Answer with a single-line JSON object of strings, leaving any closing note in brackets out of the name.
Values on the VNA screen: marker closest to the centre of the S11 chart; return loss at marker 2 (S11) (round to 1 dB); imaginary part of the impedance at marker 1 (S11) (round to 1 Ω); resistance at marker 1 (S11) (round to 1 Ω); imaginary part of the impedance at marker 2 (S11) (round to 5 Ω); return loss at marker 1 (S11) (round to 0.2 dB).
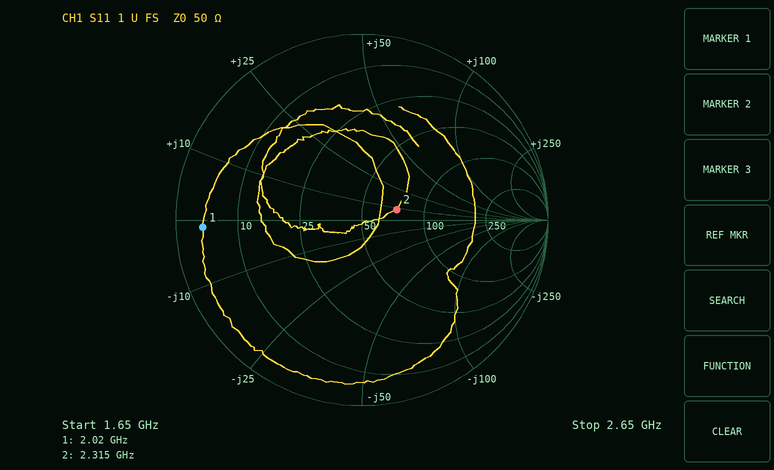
{"marker closest to the centre of the S11 chart": "marker 2", "return loss at marker 2 (S11)": "14 dB", "imaginary part of the impedance at marker 1 (S11)": "-1 Ω", "resistance at marker 1 (S11)": "4 Ω", "imaginary part of the impedance at marker 2 (S11)": "+10 Ω", "return loss at marker 1 (S11)": "1.4 dB"}
